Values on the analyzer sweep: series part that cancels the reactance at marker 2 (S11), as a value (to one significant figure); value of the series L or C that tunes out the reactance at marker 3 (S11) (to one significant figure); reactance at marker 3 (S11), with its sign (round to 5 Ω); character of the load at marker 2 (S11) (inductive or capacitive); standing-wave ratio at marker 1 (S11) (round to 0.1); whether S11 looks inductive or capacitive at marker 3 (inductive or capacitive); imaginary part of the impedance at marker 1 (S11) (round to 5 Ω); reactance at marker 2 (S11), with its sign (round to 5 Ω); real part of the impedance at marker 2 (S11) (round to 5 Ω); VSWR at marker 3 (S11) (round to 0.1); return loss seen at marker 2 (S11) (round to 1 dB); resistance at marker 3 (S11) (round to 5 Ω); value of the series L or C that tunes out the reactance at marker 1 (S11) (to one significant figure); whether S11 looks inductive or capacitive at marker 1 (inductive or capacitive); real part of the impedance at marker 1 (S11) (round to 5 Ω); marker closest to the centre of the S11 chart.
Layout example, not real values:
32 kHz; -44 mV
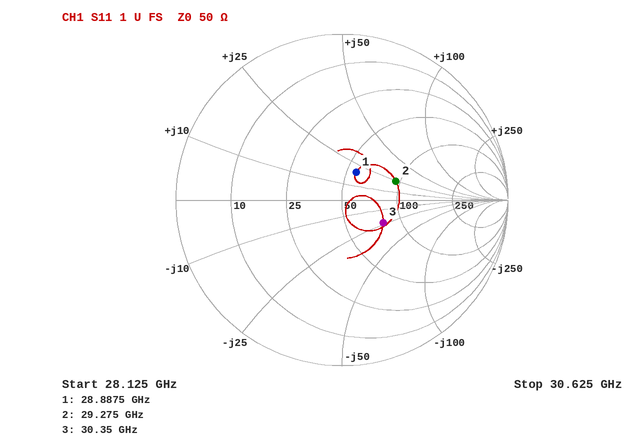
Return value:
200 fF; 100 pH; -25 Ω; inductive; 1.5; capacitive; +20 Ω; +25 Ω; 95 Ω; 1.8; 9 dB; 80 Ω; 300 fF; inductive; 55 Ω; marker 1
